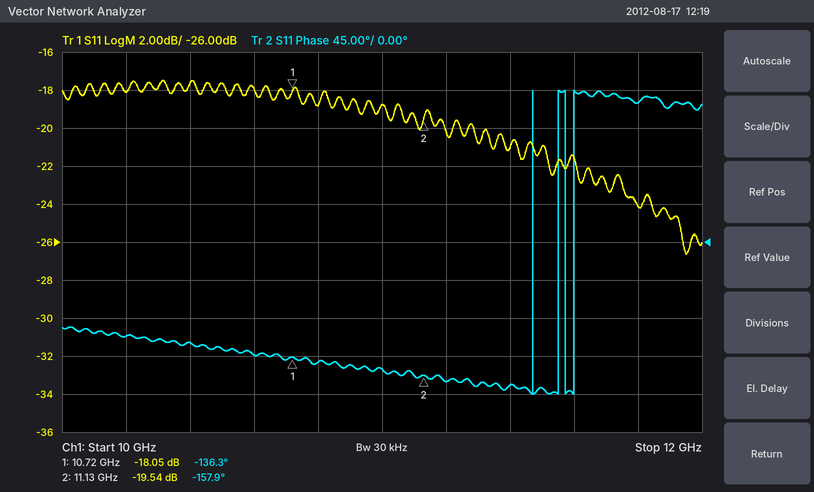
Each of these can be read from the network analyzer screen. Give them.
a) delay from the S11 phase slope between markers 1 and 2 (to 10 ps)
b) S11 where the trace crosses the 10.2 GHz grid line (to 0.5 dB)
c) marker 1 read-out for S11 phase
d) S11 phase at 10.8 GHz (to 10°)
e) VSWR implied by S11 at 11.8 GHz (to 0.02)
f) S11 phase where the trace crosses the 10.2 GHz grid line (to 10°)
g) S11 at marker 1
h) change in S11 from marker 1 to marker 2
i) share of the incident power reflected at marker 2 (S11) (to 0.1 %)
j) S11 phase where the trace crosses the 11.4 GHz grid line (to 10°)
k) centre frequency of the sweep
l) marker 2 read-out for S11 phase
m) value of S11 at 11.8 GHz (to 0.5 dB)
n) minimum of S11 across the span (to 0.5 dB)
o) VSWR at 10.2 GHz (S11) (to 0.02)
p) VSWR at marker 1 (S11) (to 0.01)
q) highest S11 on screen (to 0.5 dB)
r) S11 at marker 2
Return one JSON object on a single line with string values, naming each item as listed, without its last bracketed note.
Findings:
{"delay from the S11 phase slope between markers 1 and 2": "150 ps", "S11 where the trace crosses the 10.2 GHz grid line": "-18.0 dB", "marker 1 read-out for S11 phase": "-136.3°", "S11 phase at 10.8 GHz": "-140°", "VSWR implied by S11 at 11.8 GHz": "1.14", "S11 phase where the trace crosses the 10.2 GHz grid line": "-110°", "S11 at marker 1": "-18.05 dB", "change in S11 from marker 1 to marker 2": "-1.49 dB", "share of the incident power reflected at marker 2 (S11)": "1.1 %", "S11 phase where the trace crosses the 11.4 GHz grid line": "-170°", "centre frequency of the sweep": "11 GHz", "marker 2 read-out for S11 phase": "-157.9°", "value of S11 at 11.8 GHz": "-24.0 dB", "minimum of S11 across the span": "-26.5 dB", "VSWR at 10.2 GHz (S11)": "1.28", "VSWR at marker 1 (S11)": "1.29", "highest S11 on screen": "-17.5 dB", "S11 at marker 2": "-19.54 dB"}
